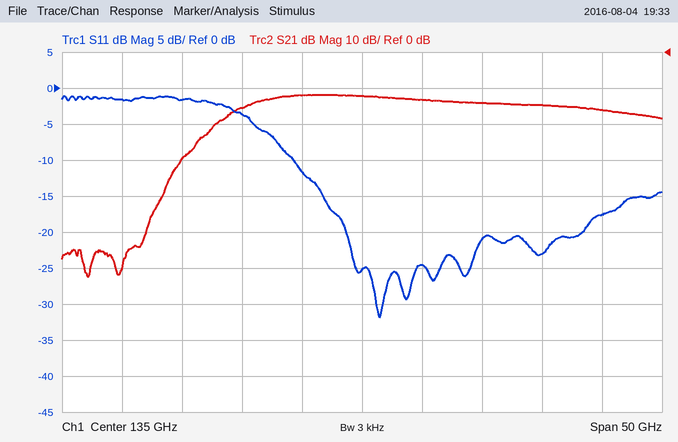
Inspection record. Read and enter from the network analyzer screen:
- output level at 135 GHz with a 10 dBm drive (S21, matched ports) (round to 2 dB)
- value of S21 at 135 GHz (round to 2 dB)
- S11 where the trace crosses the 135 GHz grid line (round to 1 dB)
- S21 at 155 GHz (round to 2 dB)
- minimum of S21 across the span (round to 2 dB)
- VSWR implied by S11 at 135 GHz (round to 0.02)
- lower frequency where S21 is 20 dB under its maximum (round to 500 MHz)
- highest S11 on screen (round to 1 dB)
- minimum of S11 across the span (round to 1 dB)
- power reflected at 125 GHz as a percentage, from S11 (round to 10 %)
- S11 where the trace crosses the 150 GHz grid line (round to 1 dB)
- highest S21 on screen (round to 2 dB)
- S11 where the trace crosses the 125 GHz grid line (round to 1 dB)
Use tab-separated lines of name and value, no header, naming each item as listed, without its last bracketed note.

output level at 135 GHz with a 10 dBm drive (S21, matched ports)	-2 dBm
value of S21 at 135 GHz	-12 dB
S11 where the trace crosses the 135 GHz grid line	-25 dB
S21 at 155 GHz	-16 dB
minimum of S21 across the span	-62 dB
VSWR implied by S11 at 135 GHz	1.12
lower frequency where S21 is 20 dB under its maximum	119.5 GHz
highest S11 on screen	-1 dB
minimum of S11 across the span	-32 dB
power reflected at 125 GHz as a percentage, from S11	40 %
S11 where the trace crosses the 150 GHz grid line	-23 dB
highest S21 on screen	-12 dB
S11 where the trace crosses the 125 GHz grid line	-4 dB
